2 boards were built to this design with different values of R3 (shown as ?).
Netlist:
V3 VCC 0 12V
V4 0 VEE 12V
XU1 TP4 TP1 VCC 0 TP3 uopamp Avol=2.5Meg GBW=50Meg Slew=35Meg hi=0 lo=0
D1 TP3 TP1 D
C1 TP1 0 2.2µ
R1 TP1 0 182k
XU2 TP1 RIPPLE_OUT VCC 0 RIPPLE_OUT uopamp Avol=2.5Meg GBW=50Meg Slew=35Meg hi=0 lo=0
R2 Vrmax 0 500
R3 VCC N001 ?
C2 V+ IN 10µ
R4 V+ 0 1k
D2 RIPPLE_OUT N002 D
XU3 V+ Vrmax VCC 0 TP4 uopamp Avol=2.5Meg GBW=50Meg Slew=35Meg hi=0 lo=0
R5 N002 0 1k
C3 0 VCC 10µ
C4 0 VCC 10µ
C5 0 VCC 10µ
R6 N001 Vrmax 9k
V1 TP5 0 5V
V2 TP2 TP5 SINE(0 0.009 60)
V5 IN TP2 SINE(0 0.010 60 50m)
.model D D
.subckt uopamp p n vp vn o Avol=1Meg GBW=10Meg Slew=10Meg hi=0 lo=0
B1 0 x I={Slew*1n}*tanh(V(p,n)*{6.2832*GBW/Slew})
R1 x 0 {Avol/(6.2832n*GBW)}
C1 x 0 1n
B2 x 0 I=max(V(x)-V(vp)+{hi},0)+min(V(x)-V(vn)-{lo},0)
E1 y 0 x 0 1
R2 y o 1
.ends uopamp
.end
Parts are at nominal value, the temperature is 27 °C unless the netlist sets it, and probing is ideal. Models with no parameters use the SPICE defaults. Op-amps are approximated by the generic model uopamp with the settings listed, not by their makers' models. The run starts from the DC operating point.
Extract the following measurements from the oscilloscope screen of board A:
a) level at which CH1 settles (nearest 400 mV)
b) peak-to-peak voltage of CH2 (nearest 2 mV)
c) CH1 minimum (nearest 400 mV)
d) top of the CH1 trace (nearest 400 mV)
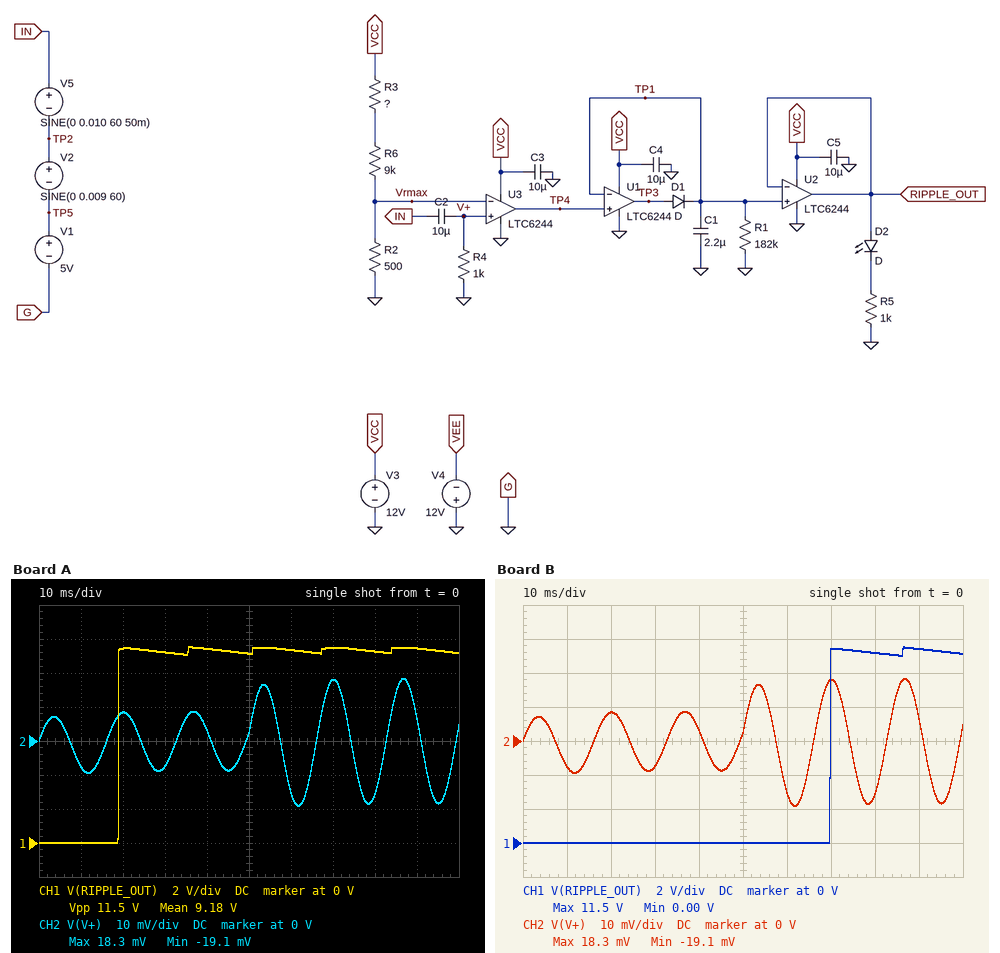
11.2 V
38 mV
0 V
11.6 V
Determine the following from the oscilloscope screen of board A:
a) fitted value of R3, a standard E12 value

820 kΩ
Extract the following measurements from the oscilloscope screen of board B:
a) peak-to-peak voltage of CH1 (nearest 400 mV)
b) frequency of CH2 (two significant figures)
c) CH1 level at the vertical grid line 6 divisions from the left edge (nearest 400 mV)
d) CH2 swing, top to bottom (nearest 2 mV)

11.6 V
60 Hz
0 V
38 mV
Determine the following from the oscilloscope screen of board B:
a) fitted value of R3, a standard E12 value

330 kΩ
